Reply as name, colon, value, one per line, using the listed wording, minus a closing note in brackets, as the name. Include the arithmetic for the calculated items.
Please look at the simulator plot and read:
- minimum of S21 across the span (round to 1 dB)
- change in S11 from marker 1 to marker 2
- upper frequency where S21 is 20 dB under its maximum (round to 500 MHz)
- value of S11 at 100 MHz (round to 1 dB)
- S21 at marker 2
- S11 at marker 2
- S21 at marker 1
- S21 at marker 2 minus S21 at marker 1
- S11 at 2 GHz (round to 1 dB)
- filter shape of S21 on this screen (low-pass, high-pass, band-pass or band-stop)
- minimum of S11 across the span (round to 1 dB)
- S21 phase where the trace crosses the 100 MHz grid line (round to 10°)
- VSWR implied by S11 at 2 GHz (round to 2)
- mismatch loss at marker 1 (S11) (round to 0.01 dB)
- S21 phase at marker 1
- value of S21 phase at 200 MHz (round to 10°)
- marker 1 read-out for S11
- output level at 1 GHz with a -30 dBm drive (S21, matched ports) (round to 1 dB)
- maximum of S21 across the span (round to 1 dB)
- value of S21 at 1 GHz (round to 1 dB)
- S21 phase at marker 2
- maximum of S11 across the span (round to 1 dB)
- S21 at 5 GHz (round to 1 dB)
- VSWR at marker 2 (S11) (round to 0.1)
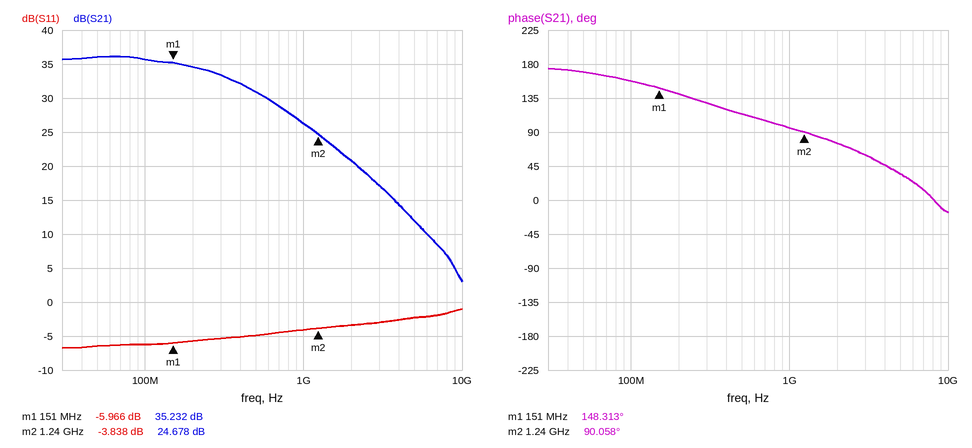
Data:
minimum of S21 across the span: 3 dB
change in S11 from marker 1 to marker 2: -3.838 − (-5.966) = 2.128 dB
upper frequency where S21 is 20 dB under its maximum: 3.5 GHz
value of S11 at 100 MHz: -6 dB
S21 at marker 2: 24.678 dB
S11 at marker 2: -3.838 dB
S21 at marker 1: 35.232 dB
S21 at marker 2 minus S21 at marker 1: 24.678 − (35.232) = -10.554 dB
S11 at 2 GHz: -3 dB
filter shape of S21 on this screen: low-pass
minimum of S11 across the span: -7 dB
S21 phase where the trace crosses the 100 MHz grid line: 160°
VSWR implied by S11 at 2 GHz: |Γ| = 10^(-3/20) = 0.7079; VSWR = (1 + 0.7079)/(1 − 0.7079) ≈ 6
mismatch loss at marker 1 (S11): −10 log10(1 − 10^(-5.966/10)) ≈ 1.27 dB
S21 phase at marker 1: 148.313°
value of S21 phase at 200 MHz: 140°
marker 1 read-out for S11: -5.966 dB
output level at 1 GHz with a -30 dBm drive (S21, matched ports): -30 dBm + (26 dB) = -4 dBm
maximum of S21 across the span: 36 dB
value of S21 at 1 GHz: 26 dB
S21 phase at marker 2: 90.058°
maximum of S11 across the span: -1 dB
S21 at 5 GHz: 12 dB
VSWR at marker 2 (S11): (1 + 0.6428)/(1 − 0.6428) ≈ 4.6
